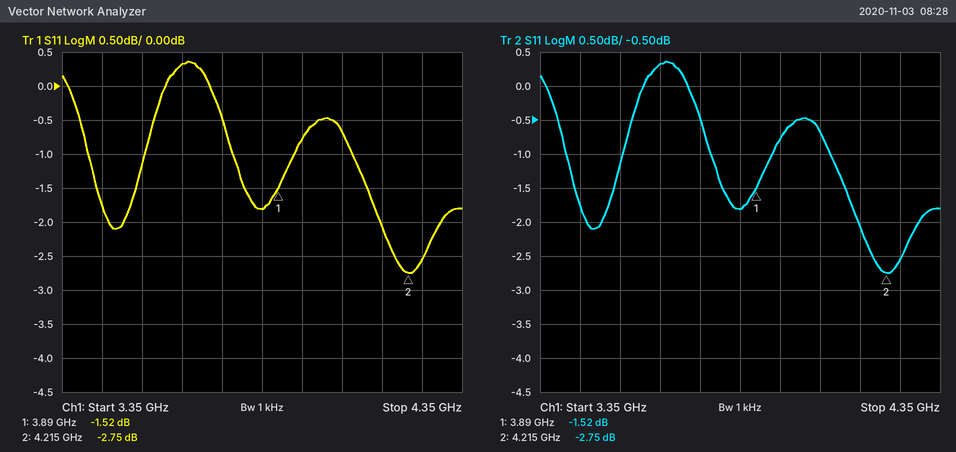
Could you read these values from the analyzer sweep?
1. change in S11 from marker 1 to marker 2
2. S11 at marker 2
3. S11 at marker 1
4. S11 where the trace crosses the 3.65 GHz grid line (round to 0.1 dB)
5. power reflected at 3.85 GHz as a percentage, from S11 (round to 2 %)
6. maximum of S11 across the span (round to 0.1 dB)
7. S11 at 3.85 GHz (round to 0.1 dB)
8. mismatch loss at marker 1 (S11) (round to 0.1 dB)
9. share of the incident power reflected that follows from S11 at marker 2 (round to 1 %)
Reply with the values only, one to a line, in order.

-1.23 dB
-2.75 dB
-1.52 dB
0.3 dB
66 %
0.4 dB
-1.8 dB
5.3 dB
53 %
